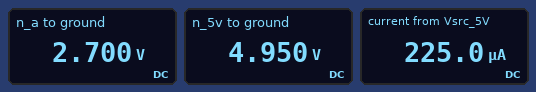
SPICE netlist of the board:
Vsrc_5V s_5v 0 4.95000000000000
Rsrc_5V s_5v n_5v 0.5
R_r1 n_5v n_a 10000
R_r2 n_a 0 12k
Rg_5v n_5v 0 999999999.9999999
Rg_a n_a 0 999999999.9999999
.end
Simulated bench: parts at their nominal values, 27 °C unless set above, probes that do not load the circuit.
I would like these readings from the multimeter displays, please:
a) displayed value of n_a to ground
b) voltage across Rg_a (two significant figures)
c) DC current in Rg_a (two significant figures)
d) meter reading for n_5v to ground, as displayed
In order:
2.700 V
2.7 V
2.7 nA
4.950 V
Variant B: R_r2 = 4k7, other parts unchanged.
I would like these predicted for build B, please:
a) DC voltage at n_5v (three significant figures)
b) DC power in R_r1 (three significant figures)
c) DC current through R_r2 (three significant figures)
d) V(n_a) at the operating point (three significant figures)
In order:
4.95 V
1.13 mW
337 µA
1.58 V
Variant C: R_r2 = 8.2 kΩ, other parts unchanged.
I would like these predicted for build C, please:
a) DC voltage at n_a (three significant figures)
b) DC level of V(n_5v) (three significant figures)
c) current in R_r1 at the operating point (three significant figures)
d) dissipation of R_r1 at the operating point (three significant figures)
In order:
2.23 V
4.95 V
272 µA
740 µW
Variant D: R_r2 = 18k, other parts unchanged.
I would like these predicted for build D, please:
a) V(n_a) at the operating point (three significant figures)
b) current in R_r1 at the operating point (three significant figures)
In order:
3.18 V
177 µA
